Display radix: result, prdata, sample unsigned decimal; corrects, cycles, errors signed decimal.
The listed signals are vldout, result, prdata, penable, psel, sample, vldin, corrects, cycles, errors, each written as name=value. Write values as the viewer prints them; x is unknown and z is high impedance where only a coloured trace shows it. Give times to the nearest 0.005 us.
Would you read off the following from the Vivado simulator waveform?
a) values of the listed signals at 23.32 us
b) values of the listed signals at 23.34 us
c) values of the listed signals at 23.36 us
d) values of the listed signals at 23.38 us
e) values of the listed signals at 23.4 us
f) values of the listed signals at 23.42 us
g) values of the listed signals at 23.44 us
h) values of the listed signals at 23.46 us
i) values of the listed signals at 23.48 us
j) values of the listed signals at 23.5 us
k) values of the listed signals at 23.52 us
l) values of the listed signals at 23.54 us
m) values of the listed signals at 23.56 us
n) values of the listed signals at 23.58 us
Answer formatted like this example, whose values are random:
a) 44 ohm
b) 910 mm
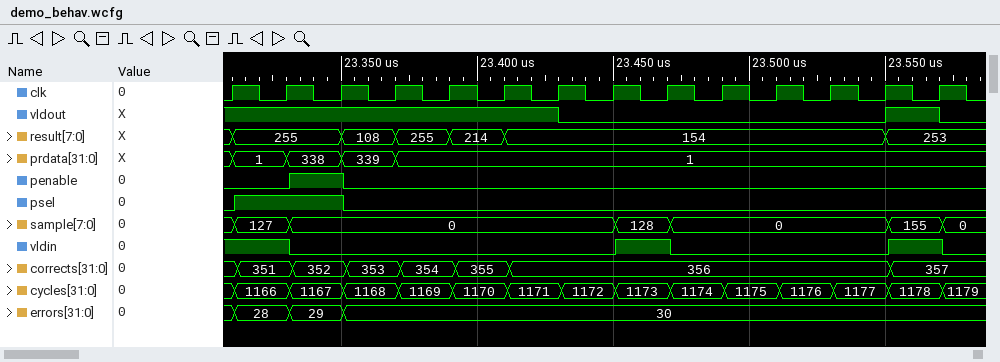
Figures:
a) vldout=1, result=255, prdata=1, penable=0, psel=1, sample=127, vldin=1, corrects=351, cycles=1166, errors=28
b) vldout=1, result=255, prdata=338, penable=1, psel=1, sample=0, vldin=0, corrects=352, cycles=1167, errors=29
c) vldout=1, result=108, prdata=339, penable=0, psel=0, sample=0, vldin=0, corrects=353, cycles=1168, errors=30
d) vldout=1, result=255, prdata=1, penable=0, psel=0, sample=0, vldin=0, corrects=354, cycles=1169, errors=30
e) vldout=1, result=214, prdata=1, penable=0, psel=0, sample=0, vldin=0, corrects=355, cycles=1170, errors=30
f) vldout=1, result=154, prdata=1, penable=0, psel=0, sample=0, vldin=0, corrects=356, cycles=1171, errors=30
g) vldout=0, result=154, prdata=1, penable=0, psel=0, sample=0, vldin=0, corrects=356, cycles=1172, errors=30
h) vldout=0, result=154, prdata=1, penable=0, psel=0, sample=128, vldin=1, corrects=356, cycles=1173, errors=30
i) vldout=0, result=154, prdata=1, penable=0, psel=0, sample=0, vldin=0, corrects=356, cycles=1174, errors=30
j) vldout=0, result=154, prdata=1, penable=0, psel=0, sample=0, vldin=0, corrects=356, cycles=1175, errors=30
k) vldout=0, result=154, prdata=1, penable=0, psel=0, sample=0, vldin=0, corrects=356, cycles=1176, errors=30
l) vldout=0, result=154, prdata=1, penable=0, psel=0, sample=0, vldin=0, corrects=356, cycles=1177, errors=30
m) vldout=1, result=253, prdata=1, penable=0, psel=0, sample=155, vldin=1, corrects=357, cycles=1178, errors=30
n) vldout=0, result=253, prdata=1, penable=0, psel=0, sample=0, vldin=0, corrects=357, cycles=1179, errors=30
